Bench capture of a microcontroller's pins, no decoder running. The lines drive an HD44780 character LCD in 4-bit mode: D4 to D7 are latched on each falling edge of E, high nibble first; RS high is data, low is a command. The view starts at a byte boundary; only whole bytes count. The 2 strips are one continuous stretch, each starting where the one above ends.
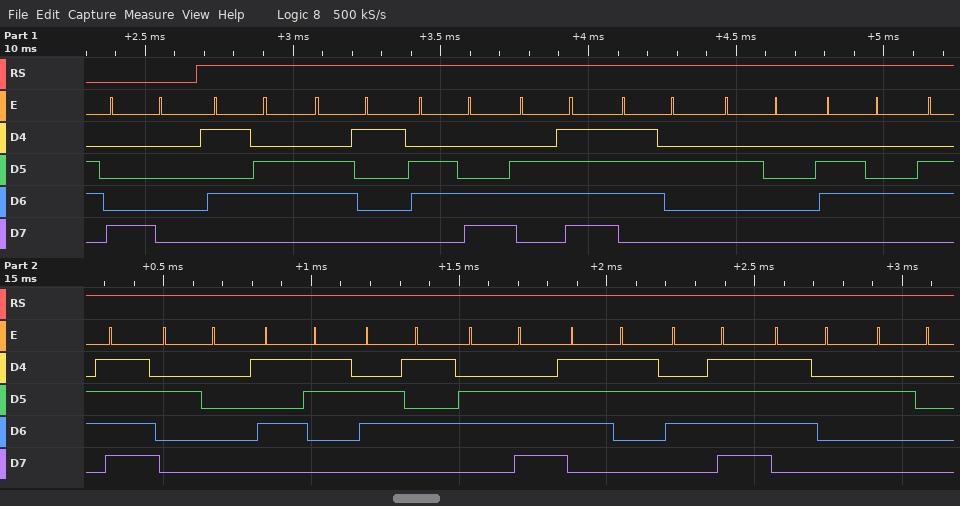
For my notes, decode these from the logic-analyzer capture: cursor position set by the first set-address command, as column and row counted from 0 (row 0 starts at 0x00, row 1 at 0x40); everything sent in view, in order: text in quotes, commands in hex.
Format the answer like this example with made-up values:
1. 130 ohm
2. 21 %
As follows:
1. column 0, row 0
2. 0x80 "Valor do Sensor "
